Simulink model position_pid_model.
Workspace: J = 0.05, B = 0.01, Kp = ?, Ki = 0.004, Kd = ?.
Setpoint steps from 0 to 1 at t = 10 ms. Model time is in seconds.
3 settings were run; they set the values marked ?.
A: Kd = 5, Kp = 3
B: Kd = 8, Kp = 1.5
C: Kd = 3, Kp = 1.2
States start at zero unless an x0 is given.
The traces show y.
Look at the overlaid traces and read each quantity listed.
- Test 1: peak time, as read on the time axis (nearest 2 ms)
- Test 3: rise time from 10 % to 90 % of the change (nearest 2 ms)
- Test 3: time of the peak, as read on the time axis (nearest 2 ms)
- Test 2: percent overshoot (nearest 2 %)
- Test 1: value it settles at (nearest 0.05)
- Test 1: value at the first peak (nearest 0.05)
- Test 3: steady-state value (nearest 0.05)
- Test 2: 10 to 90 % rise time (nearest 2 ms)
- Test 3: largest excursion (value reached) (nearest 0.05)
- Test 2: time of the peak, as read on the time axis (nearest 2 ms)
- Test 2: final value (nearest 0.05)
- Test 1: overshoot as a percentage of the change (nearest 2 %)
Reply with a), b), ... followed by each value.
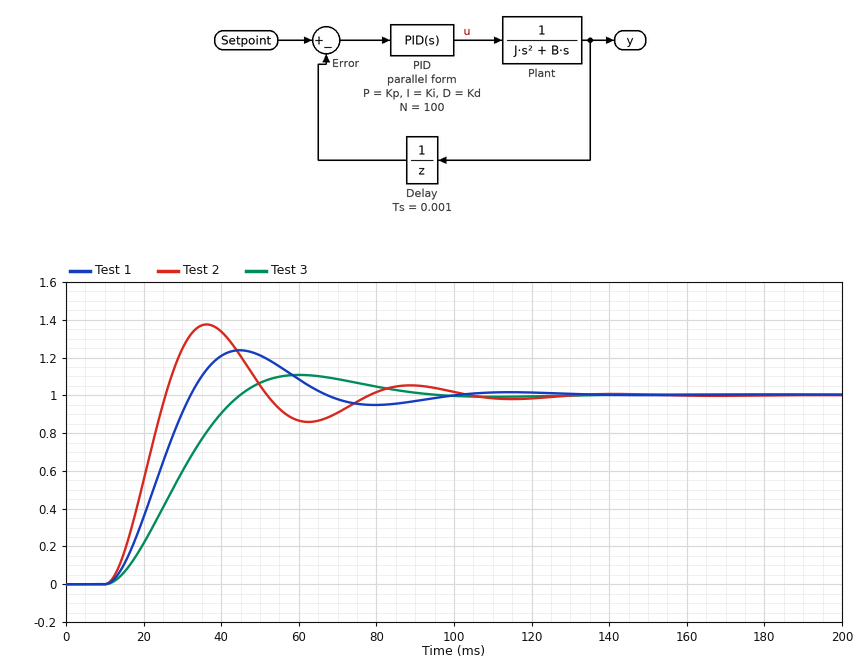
a) 44 ms
b) 24 ms
c) 60 ms
d) 38 %
e) 1.00
f) 1.25
g) 1.00
h) 10 ms
i) 1.10
j) 36 ms
k) 1.00
l) 24 %
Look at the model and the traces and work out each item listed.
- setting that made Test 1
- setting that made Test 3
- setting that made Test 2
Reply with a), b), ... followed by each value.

a) A
b) C
c) B
